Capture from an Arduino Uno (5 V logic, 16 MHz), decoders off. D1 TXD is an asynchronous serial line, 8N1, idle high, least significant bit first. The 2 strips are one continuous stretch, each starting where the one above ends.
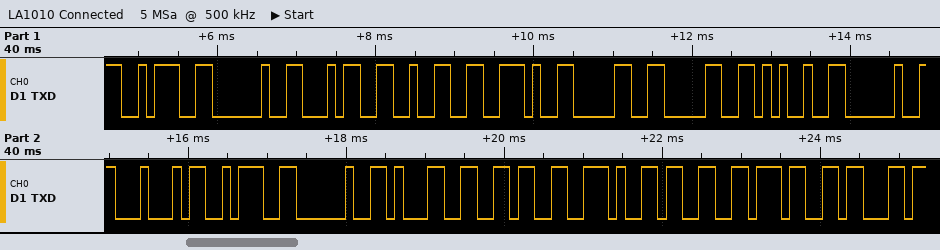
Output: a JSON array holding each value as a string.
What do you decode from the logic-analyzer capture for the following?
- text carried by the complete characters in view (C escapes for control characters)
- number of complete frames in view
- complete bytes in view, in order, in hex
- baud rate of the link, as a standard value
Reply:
["\": 42.00% D: 16.37c\"", "18", "0x3A 0x20 0x34 0x32 0x2E 0x30 0x30 0x25 0x20 0x44 0x3A 0x20 0x31 0x36 0x2E 0x33 0x37 0x63", "9600 baud"]
